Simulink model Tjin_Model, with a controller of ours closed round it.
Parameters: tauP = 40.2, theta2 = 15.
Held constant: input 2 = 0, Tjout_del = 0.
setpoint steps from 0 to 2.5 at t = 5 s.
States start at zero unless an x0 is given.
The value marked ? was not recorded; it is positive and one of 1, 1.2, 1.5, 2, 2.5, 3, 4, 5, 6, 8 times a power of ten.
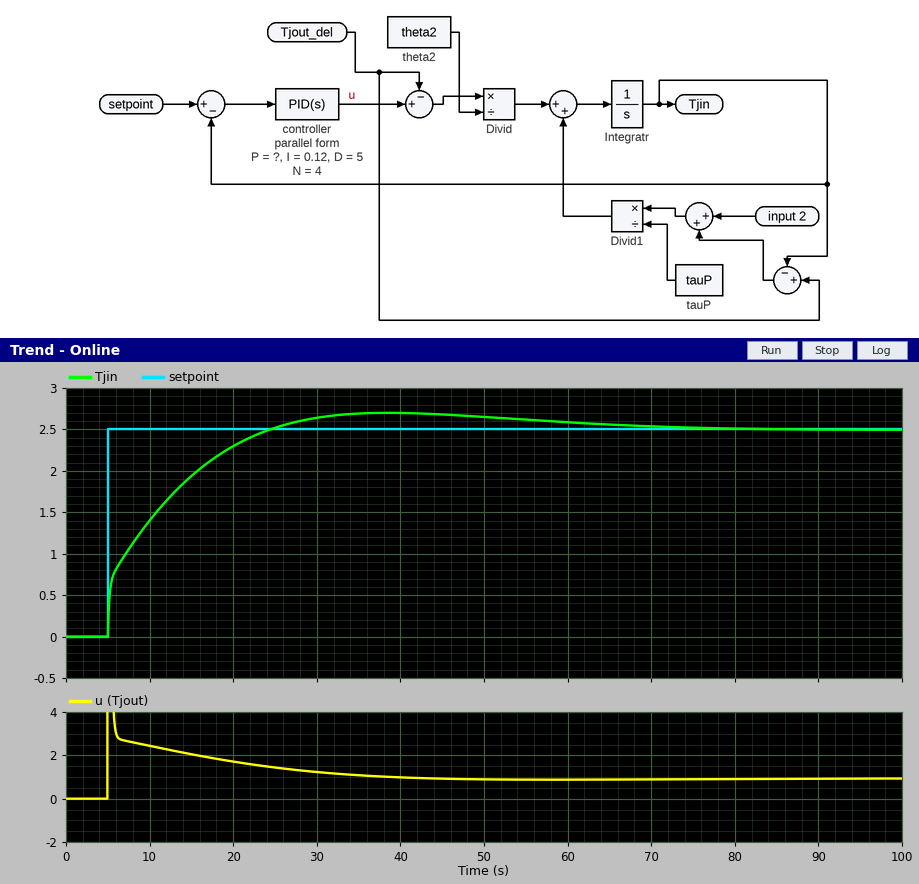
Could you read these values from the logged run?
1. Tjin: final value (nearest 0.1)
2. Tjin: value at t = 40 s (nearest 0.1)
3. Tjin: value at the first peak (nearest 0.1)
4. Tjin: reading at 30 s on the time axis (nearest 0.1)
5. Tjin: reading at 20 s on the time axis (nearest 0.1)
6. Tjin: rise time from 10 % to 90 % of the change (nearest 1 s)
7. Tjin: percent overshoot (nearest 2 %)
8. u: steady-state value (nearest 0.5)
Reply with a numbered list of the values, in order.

1. 2.5
2. 2.7
3. 2.7
4. 2.6
5. 2.3
6. 14 s
7. 8 %
8. 1.0
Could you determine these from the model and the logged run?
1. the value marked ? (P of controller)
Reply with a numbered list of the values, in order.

1. 2
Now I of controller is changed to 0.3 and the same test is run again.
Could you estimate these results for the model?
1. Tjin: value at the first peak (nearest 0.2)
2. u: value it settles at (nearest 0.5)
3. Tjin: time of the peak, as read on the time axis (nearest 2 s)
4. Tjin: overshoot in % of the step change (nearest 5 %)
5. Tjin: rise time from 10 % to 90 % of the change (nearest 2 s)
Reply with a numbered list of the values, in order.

1. 3.0
2. 1.0
3. 26 s
4. 20 %
5. 10 s
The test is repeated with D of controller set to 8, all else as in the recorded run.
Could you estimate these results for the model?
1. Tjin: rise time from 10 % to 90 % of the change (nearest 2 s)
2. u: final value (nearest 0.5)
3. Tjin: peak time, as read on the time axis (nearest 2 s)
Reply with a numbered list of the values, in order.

1. 16 s
2. 1.0
3. 42 s
